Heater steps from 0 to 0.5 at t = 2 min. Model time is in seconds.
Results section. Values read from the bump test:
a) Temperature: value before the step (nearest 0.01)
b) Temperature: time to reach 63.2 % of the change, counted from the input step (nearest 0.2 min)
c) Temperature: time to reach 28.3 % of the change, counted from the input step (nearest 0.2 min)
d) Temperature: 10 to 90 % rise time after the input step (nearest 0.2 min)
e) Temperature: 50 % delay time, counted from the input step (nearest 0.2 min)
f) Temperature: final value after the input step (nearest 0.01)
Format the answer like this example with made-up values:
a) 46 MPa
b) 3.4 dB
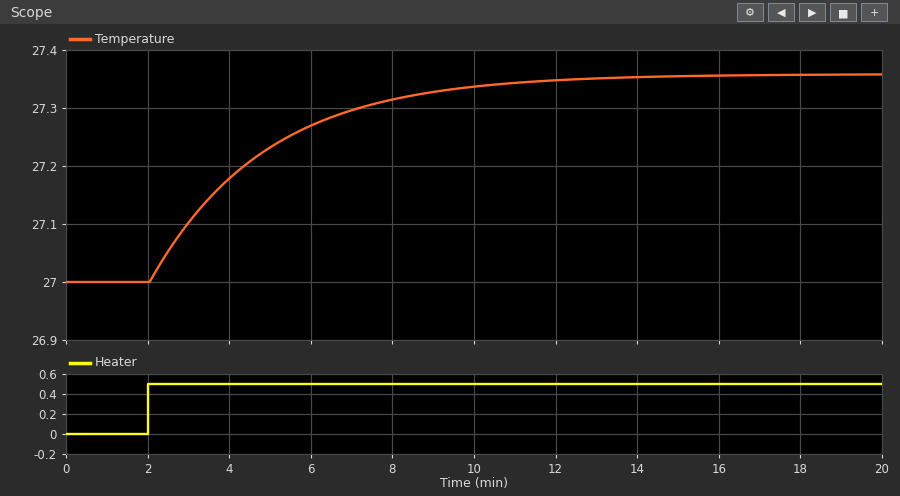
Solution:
a) 27.00
b) 2.8 min
c) 1.0 min
d) 6.2 min
e) 2.0 min
f) 27.36
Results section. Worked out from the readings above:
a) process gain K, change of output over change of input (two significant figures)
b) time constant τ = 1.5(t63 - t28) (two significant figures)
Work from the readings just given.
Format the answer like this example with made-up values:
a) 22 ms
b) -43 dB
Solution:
a) 0.72
b) 2.7 min
